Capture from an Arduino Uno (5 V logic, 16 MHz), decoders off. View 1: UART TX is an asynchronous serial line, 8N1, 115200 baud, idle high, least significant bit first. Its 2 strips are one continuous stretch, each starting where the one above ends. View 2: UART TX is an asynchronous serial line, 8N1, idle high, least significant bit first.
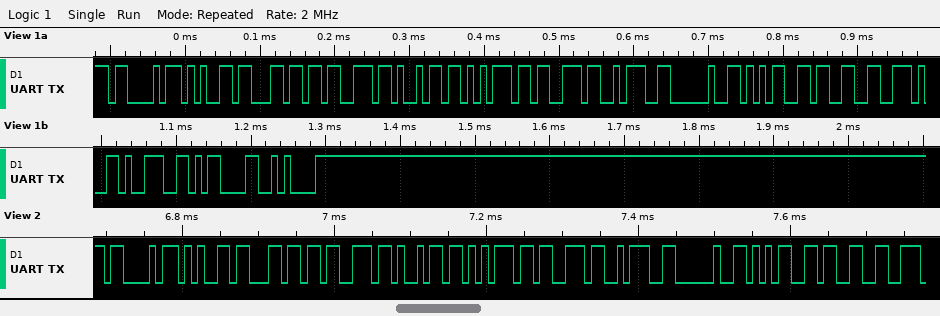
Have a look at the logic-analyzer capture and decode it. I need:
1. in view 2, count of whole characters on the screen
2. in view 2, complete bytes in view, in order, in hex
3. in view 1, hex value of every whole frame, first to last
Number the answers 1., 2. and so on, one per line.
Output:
1. 11
2. 0x43 0x65 0x6C 0x73 0x69 0x75 0x73 0x3A 0x20 0x35 0x33
3. 43 65 6C 73 69 75 73 3A 20 35 33 2E 39 0D 0A
